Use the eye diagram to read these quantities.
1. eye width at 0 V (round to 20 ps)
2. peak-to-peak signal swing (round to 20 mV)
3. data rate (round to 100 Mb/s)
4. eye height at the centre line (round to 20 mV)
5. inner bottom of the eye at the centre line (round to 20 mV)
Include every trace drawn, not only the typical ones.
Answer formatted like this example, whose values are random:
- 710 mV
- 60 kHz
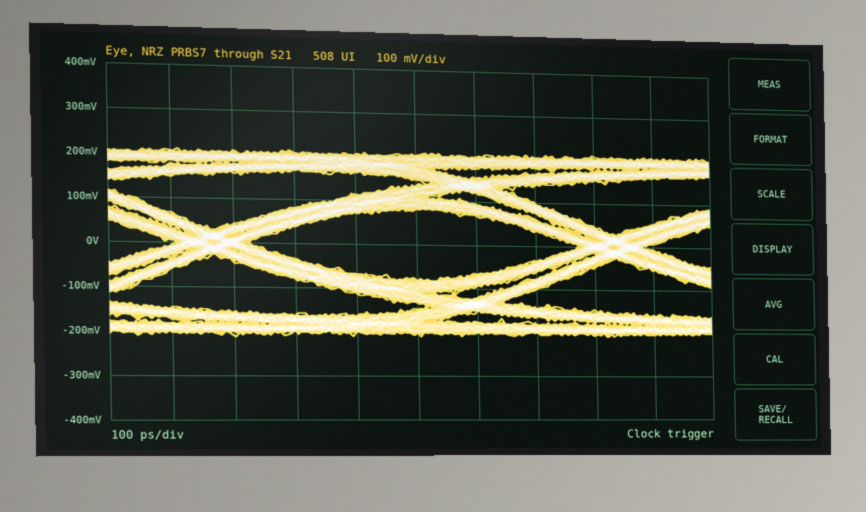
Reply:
- 540 ps
- 420 mV
- 1.5 Gb/s
- 160 mV
- -80 mV
